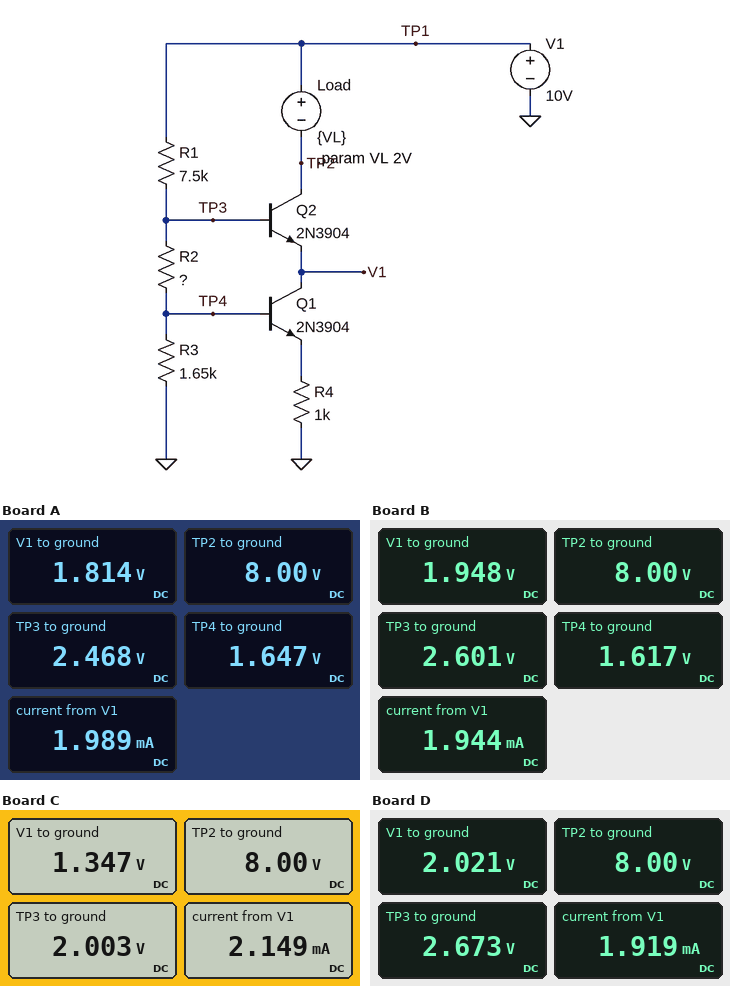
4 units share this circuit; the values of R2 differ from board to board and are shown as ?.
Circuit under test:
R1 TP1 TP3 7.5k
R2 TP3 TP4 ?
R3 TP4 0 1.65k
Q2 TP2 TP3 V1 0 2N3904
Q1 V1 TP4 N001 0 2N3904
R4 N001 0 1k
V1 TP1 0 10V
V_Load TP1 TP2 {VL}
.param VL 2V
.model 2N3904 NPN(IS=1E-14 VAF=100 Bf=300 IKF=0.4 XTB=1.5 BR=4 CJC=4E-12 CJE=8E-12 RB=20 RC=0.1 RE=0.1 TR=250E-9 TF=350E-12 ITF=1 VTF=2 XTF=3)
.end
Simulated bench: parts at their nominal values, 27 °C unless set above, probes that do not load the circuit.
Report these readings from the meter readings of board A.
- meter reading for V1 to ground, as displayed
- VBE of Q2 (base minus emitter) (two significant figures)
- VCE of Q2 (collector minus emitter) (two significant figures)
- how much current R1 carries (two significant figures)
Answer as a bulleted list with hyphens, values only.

- 1.814 V
- 650 mV
- 6.2 V
- 1.0 mA
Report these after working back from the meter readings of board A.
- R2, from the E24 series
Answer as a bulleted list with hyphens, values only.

- 820 Ω
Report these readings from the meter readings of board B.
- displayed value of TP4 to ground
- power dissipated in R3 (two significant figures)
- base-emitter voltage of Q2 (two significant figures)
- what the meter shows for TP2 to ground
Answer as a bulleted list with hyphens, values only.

- 1.617 V
- 1.6 mW
- 650 mV
- 8.00 V
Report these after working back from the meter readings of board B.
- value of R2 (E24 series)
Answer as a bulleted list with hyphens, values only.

- 1 kΩ
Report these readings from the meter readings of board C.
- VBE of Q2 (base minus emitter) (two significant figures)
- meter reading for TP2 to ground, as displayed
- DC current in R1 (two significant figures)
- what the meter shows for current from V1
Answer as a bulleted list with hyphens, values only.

- 660 mV
- 8.00 V
- 1.1 mA
- 2.149 mA
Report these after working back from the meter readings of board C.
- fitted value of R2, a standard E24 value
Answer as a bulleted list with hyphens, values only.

- 240 Ω
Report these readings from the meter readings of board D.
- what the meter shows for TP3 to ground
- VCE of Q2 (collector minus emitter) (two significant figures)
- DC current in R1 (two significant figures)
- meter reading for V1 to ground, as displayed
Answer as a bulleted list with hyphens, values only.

- 2.673 V
- 6.0 V
- 980 µA
- 2.021 V
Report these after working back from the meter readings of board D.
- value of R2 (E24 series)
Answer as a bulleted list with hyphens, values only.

- 1.1 kΩ
